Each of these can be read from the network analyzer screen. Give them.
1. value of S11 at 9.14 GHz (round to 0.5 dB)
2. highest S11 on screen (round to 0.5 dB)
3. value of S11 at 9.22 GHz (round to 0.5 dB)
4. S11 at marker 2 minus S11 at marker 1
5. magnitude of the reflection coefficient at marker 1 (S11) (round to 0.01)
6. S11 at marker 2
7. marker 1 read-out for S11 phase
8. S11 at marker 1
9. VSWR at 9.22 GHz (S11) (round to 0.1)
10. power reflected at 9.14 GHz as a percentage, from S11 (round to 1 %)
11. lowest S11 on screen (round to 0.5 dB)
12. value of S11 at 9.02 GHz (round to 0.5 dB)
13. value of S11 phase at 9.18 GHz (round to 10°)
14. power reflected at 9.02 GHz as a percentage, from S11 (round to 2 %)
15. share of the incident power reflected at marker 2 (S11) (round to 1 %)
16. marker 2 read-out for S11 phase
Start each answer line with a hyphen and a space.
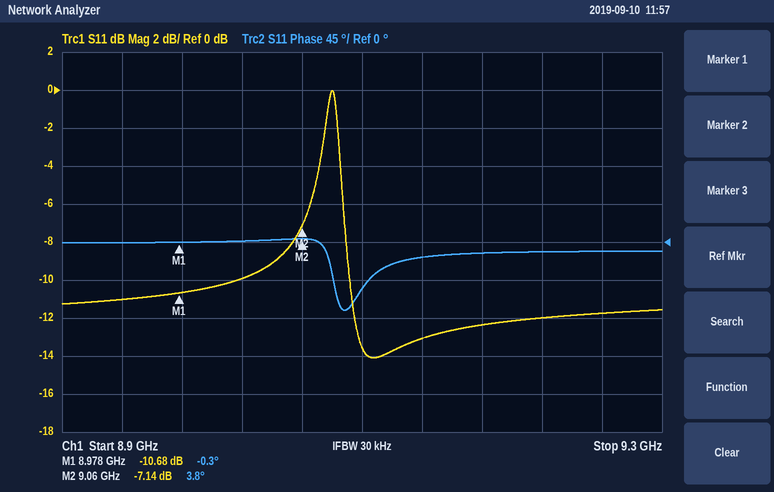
- -13.0 dB
- 0.0 dB
- -12.0 dB
- 3.54 dB
- 0.29
- -7.14 dB
- -0.3°
- -10.68 dB
- 1.7
- 5 %
- -14.0 dB
- -10.0 dB
- -10°
- 10 %
- 19 %
- 3.8°
